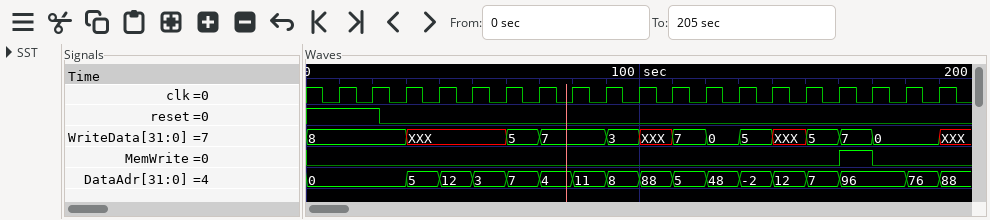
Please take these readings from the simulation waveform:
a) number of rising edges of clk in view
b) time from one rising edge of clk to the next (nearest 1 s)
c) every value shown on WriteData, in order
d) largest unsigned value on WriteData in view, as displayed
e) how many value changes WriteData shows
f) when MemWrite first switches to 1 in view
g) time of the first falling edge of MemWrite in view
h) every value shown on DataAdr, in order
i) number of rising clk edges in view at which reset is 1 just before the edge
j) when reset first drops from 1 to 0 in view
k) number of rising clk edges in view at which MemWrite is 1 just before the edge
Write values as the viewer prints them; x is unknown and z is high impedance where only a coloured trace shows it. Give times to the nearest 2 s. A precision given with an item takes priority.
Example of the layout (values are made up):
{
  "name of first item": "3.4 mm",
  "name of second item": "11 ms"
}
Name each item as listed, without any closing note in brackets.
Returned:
{
  "number of rising edges of clk in view": "19",
  "time from one rising edge of clk to the next": "10 s",
  "every value shown on WriteData, in order": "8, XXX, 5, 7, 3, XXX, 7, 0, 5, XXX, 5, 7, 0, XXX",
  "largest unsigned value on WriteData in view, as displayed": "8",
  "how many value changes WriteData shows": "13",
  "when MemWrite first switches to 1 in view": "160 s",
  "time of the first falling edge of MemWrite in view": "170 s",
  "every value shown on DataAdr, in order": "0, 5, 12, 3, 7, 4, 11, 8, 88, 5, 48, -2, 12, 7, 96, 76, 88",
  "number of rising clk edges in view at which reset is 1 just before the edge": "2",
  "when reset first drops from 1 to 0 in view": "22 s",
  "number of rising clk edges in view at which MemWrite is 1 just before the edge": "1"
}
